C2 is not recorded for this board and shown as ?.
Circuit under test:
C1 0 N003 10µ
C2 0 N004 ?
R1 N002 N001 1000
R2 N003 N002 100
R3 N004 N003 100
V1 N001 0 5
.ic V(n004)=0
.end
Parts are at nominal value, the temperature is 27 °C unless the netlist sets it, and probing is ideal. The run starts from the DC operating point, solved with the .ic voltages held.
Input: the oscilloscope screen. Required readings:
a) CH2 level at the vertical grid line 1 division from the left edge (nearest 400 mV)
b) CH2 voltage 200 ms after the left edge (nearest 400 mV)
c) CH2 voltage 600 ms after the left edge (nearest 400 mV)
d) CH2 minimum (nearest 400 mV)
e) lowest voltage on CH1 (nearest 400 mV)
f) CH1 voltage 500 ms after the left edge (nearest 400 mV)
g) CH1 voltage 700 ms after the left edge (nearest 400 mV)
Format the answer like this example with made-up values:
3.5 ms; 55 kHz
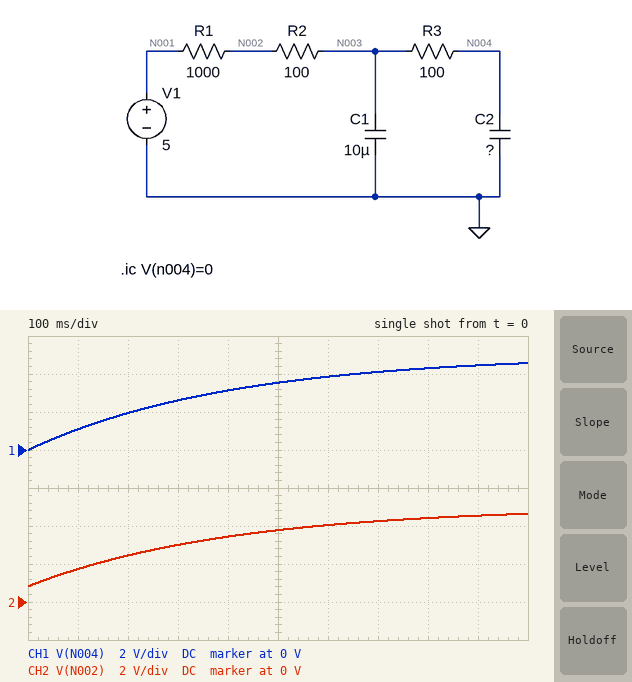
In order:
1.6 V; 2.4 V; 4.0 V; 800 mV; 0 V; 3.6 V; 4.0 V
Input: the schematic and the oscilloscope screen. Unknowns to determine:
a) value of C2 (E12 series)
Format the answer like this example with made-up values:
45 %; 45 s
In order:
330 µF
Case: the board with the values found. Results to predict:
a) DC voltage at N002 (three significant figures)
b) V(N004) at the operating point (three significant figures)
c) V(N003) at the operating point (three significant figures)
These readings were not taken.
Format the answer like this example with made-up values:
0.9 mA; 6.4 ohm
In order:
5.00 V; 5.00 V; 5.00 V
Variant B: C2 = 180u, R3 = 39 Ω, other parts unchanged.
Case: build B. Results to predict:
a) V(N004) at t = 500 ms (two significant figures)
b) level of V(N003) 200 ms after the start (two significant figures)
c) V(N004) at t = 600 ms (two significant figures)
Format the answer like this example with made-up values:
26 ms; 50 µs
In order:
4.5 V; 3.1 V; 4.7 V
